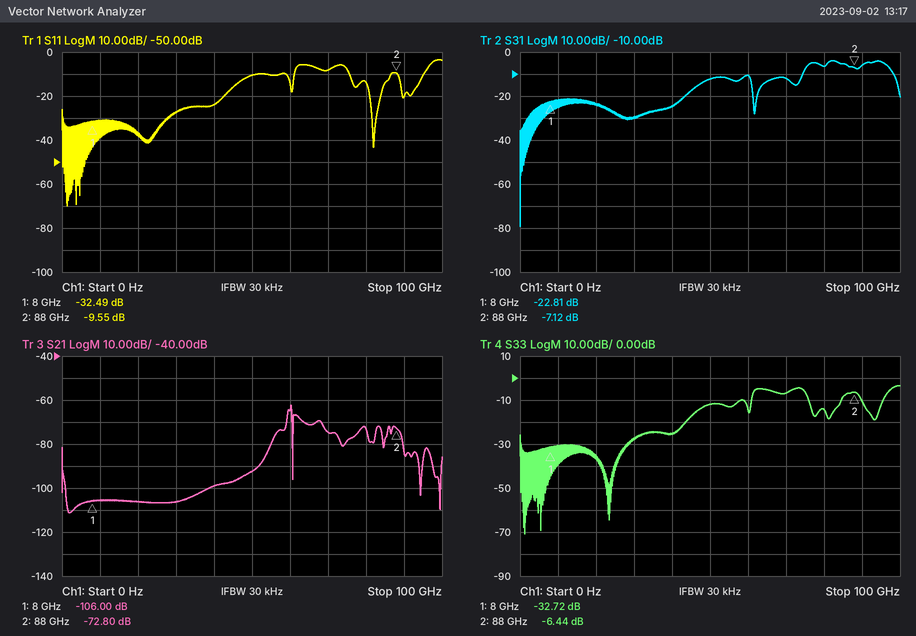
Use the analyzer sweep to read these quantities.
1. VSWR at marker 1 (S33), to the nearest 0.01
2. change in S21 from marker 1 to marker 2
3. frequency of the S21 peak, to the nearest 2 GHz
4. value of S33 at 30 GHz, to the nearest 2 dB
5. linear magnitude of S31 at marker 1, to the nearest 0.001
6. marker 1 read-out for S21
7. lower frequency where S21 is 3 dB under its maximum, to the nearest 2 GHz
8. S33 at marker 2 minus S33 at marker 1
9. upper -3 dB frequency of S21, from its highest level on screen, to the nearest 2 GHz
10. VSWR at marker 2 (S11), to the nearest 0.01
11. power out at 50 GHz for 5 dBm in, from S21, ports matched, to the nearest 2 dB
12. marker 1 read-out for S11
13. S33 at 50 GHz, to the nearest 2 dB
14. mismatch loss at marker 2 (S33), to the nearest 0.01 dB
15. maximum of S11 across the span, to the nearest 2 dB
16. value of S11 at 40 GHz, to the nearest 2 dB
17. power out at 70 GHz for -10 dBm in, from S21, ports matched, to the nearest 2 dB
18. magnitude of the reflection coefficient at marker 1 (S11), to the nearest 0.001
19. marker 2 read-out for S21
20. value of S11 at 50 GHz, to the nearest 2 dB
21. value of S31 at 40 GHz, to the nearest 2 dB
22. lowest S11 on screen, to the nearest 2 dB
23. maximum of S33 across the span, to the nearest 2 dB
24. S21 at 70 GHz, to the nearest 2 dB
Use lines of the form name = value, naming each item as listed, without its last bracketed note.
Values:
VSWR at marker 1 (S33), to the nearest 0.01 = 1.05
change in S21 from marker 1 to marker 2 = 33.20 dB
frequency of the S21 peak, to the nearest 2 GHz = 60 GHz
value of S33 at 30 GHz, to the nearest 2 dB = -28 dB
linear magnitude of S31 at marker 1, to the nearest 0.001 = 0.072
marker 1 read-out for S21 = -106.00 dB
lower frequency where S21 is 3 dB under its maximum, to the nearest 2 GHz = 60 GHz
S33 at marker 2 minus S33 at marker 1 = 26.28 dB
upper -3 dB frequency of S21, from its highest level on screen, to the nearest 2 GHz = 60 GHz
VSWR at marker 2 (S11), to the nearest 0.01 = 2.00
power out at 50 GHz for 5 dBm in, from S21, ports matched, to the nearest 2 dB = -88 dBm
marker 1 read-out for S11 = -32.49 dB
S33 at 50 GHz, to the nearest 2 dB = -12 dB
mismatch loss at marker 2 (S33), to the nearest 0.01 dB = 1.12 dB
maximum of S11 across the span, to the nearest 2 dB = -4 dB
value of S11 at 40 GHz, to the nearest 2 dB = -24 dB
power out at 70 GHz for -10 dBm in, from S21, ports matched, to the nearest 2 dB = -84 dBm
magnitude of the reflection coefficient at marker 1 (S11), to the nearest 0.001 = 0.024
marker 2 read-out for S21 = -72.80 dB
value of S11 at 50 GHz, to the nearest 2 dB = -10 dB
value of S31 at 40 GHz, to the nearest 2 dB = -24 dB
lowest S11 on screen, to the nearest 2 dB = -70 dB
maximum of S33 across the span, to the nearest 2 dB = -4 dB
S21 at 70 GHz, to the nearest 2 dB = -74 dB
